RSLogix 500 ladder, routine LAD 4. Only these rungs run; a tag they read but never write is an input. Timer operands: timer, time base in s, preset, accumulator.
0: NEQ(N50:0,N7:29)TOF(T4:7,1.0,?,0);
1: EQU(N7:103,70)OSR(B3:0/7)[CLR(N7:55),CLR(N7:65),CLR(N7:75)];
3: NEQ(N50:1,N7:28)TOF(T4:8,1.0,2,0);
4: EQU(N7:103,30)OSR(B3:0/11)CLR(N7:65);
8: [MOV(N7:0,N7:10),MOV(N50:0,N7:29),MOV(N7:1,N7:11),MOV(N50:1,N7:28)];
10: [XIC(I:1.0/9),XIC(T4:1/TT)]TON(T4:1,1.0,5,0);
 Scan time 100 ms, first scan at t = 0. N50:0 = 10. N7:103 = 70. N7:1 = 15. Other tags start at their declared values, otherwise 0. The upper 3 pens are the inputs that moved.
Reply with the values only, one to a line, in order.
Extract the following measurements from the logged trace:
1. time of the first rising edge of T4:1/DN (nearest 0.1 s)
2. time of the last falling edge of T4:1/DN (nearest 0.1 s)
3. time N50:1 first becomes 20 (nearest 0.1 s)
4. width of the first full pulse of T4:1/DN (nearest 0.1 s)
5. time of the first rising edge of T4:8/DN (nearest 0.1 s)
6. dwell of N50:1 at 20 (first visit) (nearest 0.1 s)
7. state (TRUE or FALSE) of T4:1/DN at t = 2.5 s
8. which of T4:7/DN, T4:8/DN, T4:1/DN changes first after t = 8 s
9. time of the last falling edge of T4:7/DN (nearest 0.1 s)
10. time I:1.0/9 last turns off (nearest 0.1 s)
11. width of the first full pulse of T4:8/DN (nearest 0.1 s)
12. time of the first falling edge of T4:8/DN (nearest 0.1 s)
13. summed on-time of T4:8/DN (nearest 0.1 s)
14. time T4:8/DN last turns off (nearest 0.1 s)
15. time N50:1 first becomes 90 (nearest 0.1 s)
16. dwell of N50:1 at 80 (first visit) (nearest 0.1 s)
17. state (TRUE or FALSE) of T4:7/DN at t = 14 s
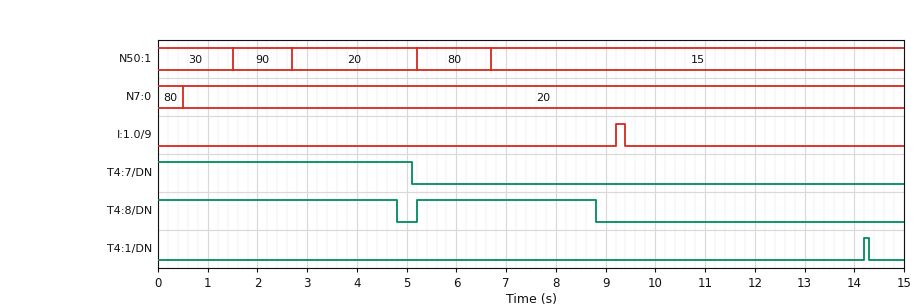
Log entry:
14.2 s
14.3 s
2.7 s
0.1 s
5.2 s
2.5 s
FALSE
T4:8/DN
5.1 s
9.4 s
3.6 s
4.8 s
8.4 s
8.8 s
1.5 s
1.5 s
FALSE
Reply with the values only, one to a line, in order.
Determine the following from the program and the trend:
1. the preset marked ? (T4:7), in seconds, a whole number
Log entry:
5 s
